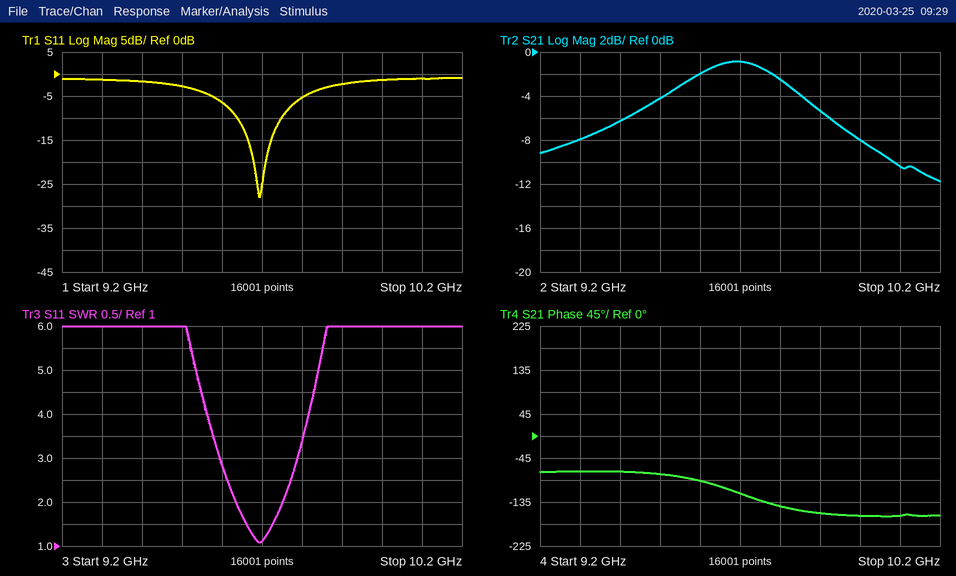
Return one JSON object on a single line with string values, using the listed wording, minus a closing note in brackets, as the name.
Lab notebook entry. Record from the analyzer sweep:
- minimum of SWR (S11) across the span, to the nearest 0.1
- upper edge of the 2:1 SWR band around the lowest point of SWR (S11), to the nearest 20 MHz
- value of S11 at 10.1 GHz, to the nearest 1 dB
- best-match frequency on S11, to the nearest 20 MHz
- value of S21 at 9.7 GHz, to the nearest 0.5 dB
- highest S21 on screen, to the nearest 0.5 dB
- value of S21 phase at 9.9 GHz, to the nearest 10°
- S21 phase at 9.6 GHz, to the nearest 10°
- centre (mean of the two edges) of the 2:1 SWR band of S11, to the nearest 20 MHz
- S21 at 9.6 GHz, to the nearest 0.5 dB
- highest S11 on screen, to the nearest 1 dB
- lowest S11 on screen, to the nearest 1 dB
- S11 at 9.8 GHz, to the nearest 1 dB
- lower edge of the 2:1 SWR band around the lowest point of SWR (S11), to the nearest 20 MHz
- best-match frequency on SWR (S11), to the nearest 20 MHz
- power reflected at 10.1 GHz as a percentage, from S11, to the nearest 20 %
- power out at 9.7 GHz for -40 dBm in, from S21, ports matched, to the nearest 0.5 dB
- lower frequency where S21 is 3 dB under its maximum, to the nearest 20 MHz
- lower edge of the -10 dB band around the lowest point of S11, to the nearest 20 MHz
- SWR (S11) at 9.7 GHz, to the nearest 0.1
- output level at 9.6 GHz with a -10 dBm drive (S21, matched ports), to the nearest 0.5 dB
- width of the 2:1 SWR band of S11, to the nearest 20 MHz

{"minimum of SWR (S11) across the span, to the nearest 0.1": "1.1", "upper edge of the 2:1 SWR band around the lowest point of SWR (S11), to the nearest 20 MHz": "9.76 GHz", "value of S11 at 10.1 GHz, to the nearest 1 dB": "-1 dB", "best-match frequency on S11, to the nearest 20 MHz": "9.70 GHz", "value of S21 at 9.7 GHz, to the nearest 0.5 dB": "-1.0 dB", "highest S21 on screen, to the nearest 0.5 dB": "-1.0 dB", "value of S21 phase at 9.9 GHz, to the nearest 10°": "-160°", "S21 phase at 9.6 GHz, to the nearest 10°": "-90°", "centre (mean of the two edges) of the 2:1 SWR band of S11, to the nearest 20 MHz": "9.70 GHz", "S21 at 9.6 GHz, to the nearest 0.5 dB": "-2.0 dB", "highest S11 on screen, to the nearest 1 dB": "-1 dB", "lowest S11 on screen, to the nearest 1 dB": "-28 dB", "S11 at 9.8 GHz, to the nearest 1 dB": "-5 dB", "lower edge of the 2:1 SWR band around the lowest point of SWR (S11), to the nearest 20 MHz": "9.64 GHz", "best-match frequency on SWR (S11), to the nearest 20 MHz": "9.70 GHz", "power reflected at 10.1 GHz as a percentage, from S11, to the nearest 20 %": "80 %", "power out at 9.7 GHz for -40 dBm in, from S21, ports matched, to the nearest 0.5 dB": "-41.0 dBm", "lower frequency where S21 is 3 dB under its maximum, to the nearest 20 MHz": "9.52 GHz", "lower edge of the -10 dB band around the lowest point of S11, to the nearest 20 MHz": "9.64 GHz", "SWR (S11) at 9.7 GHz, to the nearest 0.1": "1.1", "output level at 9.6 GHz with a -10 dBm drive (S21, matched ports), to the nearest 0.5 dB": "-12.0 dBm", "width of the 2:1 SWR band of S11, to the nearest 20 MHz": "120 MHz"}
